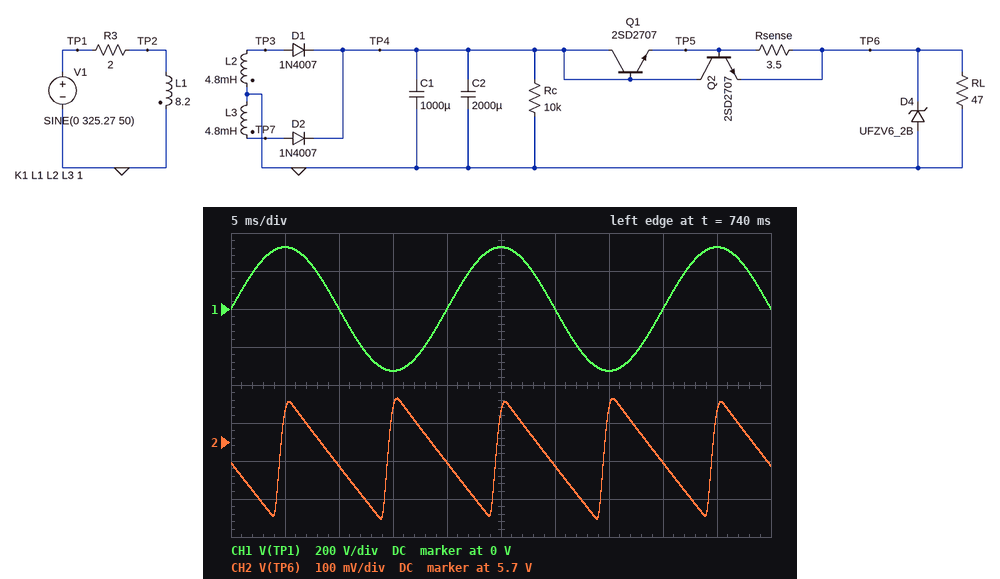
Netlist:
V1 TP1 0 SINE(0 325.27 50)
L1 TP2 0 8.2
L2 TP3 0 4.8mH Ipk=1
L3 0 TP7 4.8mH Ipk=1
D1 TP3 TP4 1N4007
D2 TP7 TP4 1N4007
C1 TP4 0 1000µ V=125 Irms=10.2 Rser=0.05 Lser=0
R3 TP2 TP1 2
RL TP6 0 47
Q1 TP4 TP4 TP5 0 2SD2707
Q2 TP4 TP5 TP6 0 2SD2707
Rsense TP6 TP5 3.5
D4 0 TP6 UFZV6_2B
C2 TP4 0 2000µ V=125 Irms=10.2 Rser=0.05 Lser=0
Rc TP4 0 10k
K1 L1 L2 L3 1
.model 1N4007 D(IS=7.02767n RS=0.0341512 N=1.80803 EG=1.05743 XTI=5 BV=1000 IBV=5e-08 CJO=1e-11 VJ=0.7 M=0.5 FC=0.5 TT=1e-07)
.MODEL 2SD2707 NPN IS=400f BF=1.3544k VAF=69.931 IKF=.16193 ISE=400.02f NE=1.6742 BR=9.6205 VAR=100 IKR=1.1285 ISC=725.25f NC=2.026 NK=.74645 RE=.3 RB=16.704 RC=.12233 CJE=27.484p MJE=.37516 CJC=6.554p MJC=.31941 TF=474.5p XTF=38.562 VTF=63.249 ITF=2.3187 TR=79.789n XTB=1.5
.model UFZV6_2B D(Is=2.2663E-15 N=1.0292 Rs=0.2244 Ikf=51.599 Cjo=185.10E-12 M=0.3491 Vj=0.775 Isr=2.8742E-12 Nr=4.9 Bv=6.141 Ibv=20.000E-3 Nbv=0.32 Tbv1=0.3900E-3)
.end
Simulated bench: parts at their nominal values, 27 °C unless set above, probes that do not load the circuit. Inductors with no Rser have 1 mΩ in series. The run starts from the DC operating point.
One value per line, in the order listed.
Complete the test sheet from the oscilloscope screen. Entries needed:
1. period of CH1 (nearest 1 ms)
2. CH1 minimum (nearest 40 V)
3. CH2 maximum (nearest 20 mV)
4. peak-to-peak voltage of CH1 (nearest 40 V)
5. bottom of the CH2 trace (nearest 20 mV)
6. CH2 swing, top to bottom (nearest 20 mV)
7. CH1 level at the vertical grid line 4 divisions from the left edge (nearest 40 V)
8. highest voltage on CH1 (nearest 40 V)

20 ms
-320 V
5.82 V
640 V
5.50 V
320 mV
0 V
320 V
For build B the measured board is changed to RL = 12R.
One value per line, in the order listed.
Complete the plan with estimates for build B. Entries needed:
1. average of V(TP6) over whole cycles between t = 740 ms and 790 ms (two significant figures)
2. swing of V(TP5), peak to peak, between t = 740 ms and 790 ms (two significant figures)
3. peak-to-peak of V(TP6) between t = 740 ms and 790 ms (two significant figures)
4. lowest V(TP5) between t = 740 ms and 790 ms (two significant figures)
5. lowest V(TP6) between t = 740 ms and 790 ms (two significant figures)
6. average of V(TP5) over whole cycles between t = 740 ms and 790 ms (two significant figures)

4.8 V
1.0 V
950 mV
5.1 V
4.3 V
5.6 V
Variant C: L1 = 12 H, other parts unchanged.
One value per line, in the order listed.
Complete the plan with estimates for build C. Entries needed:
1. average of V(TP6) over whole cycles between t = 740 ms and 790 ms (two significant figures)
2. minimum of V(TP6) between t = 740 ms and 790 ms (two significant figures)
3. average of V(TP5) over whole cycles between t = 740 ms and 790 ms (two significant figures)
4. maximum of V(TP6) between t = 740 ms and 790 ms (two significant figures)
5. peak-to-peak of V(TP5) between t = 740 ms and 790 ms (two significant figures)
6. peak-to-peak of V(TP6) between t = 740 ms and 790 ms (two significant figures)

4.5 V
4.3 V
4.8 V
4.6 V
260 mV
250 mV
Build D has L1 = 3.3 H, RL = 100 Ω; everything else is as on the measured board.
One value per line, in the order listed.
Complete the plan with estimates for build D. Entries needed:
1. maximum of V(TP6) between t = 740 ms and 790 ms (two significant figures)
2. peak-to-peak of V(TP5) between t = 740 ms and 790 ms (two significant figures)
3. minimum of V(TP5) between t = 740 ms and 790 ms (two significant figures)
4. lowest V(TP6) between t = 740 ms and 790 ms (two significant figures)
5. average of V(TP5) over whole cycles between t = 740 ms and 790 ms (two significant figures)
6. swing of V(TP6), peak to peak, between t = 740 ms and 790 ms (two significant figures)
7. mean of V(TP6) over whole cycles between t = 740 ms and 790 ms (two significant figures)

6.5 V
1.1 V
7.6 V
6.3 V
8.2 V
120 mV
6.4 V
